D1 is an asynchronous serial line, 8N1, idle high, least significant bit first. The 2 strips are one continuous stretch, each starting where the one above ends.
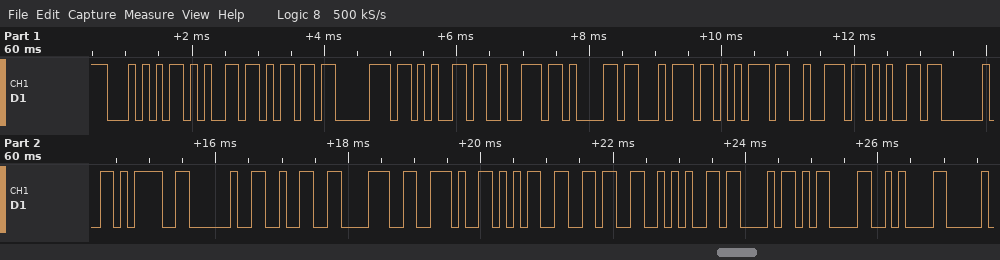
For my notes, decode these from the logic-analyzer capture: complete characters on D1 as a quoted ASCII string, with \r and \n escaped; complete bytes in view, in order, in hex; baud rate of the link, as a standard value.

"Temperature = 28.56*C\r\n"
54 65 6D 70 65 72 61 74 75 72 65 20 3D 20 32 38 2E 35 36 2A 43 0D 0A
9600 baud
